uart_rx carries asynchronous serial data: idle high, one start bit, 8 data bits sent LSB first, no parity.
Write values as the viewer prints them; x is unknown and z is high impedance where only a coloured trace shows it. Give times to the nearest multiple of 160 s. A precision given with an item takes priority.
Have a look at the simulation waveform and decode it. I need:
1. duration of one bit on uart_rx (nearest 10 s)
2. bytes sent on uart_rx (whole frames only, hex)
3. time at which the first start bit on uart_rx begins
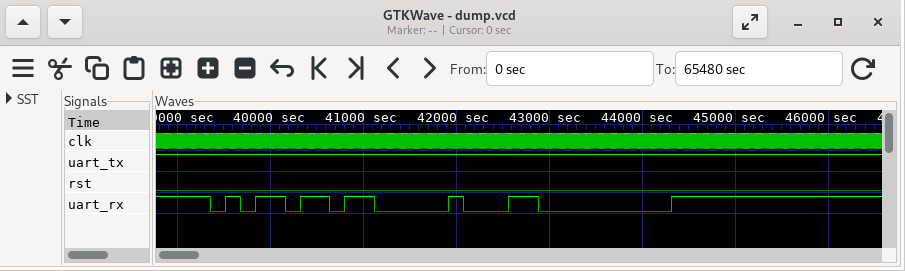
160 s
6D, 10, 00
39360 s
